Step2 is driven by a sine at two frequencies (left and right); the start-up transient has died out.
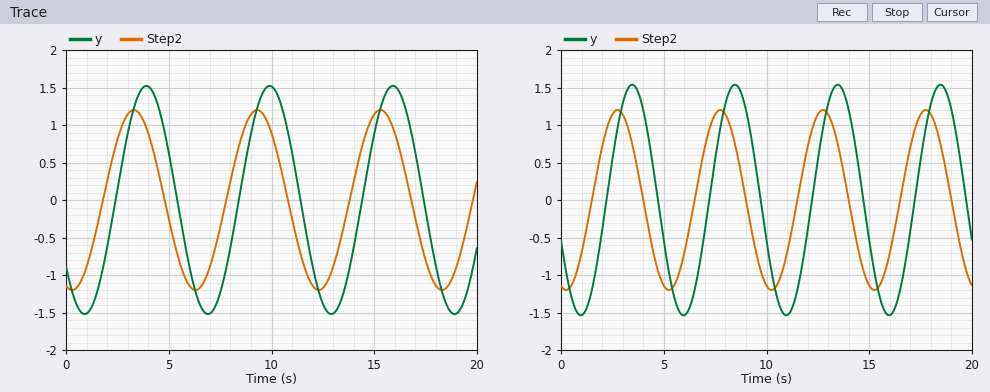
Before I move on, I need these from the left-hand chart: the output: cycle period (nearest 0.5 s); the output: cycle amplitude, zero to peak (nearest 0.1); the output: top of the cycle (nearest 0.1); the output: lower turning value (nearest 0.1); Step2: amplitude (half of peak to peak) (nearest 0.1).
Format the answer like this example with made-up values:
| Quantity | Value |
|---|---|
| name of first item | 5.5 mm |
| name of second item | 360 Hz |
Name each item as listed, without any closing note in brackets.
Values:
| Quantity | Value |
|---|---|
| the output: cycle period | 6.0 s |
| the output: cycle amplitude, zero to peak | 1.5 |
| the output: top of the cycle | 1.5 |
| the output: lower turning value | -1.5 |
| Step2: amplitude (half of peak to peak) | 1.2 |
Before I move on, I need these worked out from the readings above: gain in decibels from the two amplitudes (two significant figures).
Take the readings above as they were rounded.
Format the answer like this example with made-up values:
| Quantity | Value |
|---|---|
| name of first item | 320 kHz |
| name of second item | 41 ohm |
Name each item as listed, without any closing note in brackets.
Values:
| Quantity | Value |
|---|---|
| gain in decibels from the two amplitudes | 1.9 dB |
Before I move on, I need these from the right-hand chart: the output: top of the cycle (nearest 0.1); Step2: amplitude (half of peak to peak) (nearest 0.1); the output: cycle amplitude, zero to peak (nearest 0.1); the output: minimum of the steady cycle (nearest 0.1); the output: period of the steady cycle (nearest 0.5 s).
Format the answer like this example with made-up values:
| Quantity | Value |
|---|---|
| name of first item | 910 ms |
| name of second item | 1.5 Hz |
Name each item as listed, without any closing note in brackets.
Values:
| Quantity | Value |
|---|---|
| the output: top of the cycle | 1.5 |
| Step2: amplitude (half of peak to peak) | 1.2 |
| the output: cycle amplitude, zero to peak | 1.5 |
| the output: minimum of the steady cycle | -1.5 |
| the output: period of the steady cycle | 5.0 s |
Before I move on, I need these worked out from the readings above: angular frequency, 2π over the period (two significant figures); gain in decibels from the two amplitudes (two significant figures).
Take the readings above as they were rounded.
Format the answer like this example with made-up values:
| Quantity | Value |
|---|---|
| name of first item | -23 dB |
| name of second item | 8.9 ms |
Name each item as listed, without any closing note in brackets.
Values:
| Quantity | Value |
|---|---|
| angular frequency, 2π over the period | 1.3 rad/s |
| gain in decibels from the two amplitudes | 1.9 dB |
